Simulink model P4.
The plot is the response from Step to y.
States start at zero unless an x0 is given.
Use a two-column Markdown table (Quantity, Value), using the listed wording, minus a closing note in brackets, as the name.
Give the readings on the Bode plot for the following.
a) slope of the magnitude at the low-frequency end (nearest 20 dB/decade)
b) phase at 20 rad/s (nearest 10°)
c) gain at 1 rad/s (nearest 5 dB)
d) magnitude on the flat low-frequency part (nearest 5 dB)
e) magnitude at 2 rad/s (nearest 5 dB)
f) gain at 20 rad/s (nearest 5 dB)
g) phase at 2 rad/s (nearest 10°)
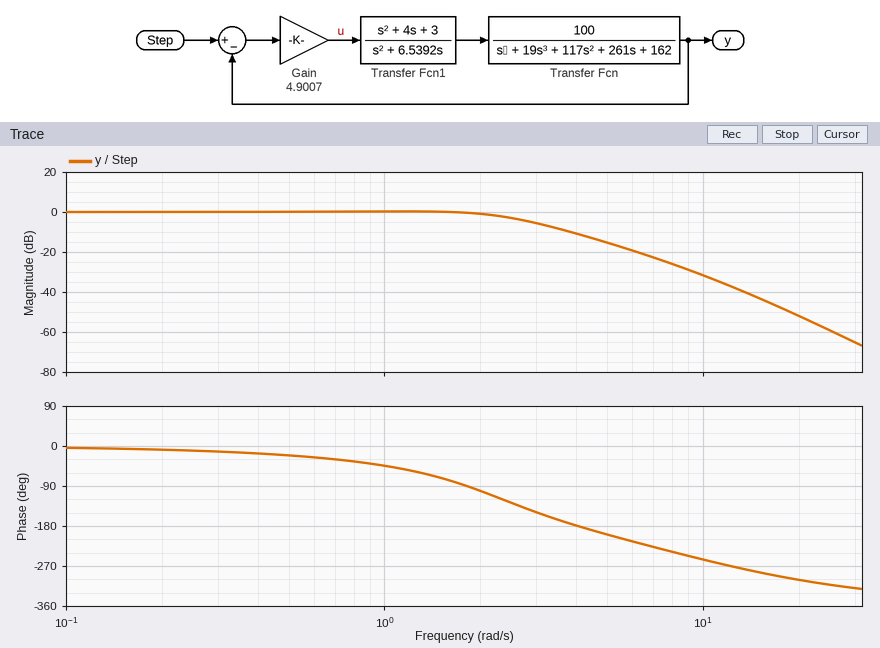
| Quantity | Value |
|---|---|
| slope of the magnitude at the low-frequency end | 0 dB/decade |
| phase at 20 rad/s | -300° |
| gain at 1 rad/s | 0 dB |
| magnitude on the flat low-frequency part | 0 dB |
| magnitude at 2 rad/s | 0 dB |
| gain at 20 rad/s | -50 dB |
| phase at 2 rad/s | -100° |
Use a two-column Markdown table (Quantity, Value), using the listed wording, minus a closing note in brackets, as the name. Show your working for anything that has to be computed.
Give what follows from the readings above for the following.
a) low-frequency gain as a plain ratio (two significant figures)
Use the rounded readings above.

| Quantity | Value |
|---|---|
| low-frequency gain as a plain ratio | 10^(0 / 20) = 1.0 |
